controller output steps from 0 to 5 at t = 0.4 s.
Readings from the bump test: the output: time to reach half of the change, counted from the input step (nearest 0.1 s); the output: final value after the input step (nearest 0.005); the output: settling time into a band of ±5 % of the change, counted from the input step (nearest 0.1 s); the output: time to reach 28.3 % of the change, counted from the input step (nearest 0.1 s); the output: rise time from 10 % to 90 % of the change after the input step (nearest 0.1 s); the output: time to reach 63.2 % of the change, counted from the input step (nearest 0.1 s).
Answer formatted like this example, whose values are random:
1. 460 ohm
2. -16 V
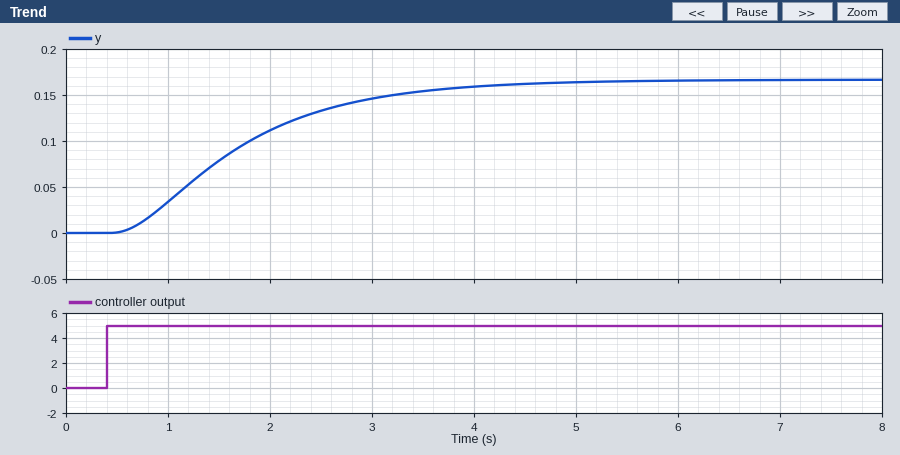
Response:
1. 1.2 s
2. 0.165
3. 3.5 s
4. 0.7 s
5. 2.4 s
6. 1.5 s
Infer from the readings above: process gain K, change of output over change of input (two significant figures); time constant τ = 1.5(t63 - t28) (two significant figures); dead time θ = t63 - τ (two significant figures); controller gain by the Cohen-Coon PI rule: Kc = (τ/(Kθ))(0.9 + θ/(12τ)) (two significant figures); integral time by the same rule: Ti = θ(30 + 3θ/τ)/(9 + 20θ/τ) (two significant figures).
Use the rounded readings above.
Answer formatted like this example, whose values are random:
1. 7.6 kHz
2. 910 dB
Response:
1. 0.033
2. 1.2 s
3. 0.30 s
4. 110
5. 0.66 s
